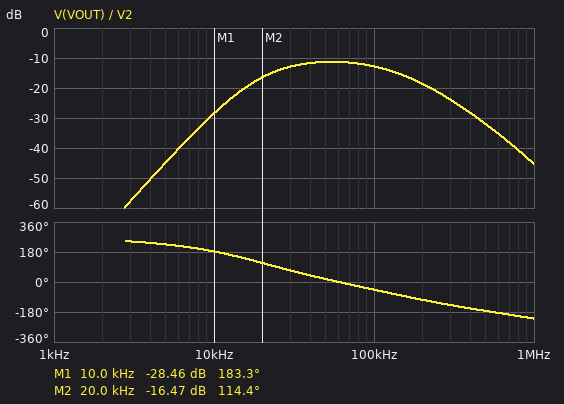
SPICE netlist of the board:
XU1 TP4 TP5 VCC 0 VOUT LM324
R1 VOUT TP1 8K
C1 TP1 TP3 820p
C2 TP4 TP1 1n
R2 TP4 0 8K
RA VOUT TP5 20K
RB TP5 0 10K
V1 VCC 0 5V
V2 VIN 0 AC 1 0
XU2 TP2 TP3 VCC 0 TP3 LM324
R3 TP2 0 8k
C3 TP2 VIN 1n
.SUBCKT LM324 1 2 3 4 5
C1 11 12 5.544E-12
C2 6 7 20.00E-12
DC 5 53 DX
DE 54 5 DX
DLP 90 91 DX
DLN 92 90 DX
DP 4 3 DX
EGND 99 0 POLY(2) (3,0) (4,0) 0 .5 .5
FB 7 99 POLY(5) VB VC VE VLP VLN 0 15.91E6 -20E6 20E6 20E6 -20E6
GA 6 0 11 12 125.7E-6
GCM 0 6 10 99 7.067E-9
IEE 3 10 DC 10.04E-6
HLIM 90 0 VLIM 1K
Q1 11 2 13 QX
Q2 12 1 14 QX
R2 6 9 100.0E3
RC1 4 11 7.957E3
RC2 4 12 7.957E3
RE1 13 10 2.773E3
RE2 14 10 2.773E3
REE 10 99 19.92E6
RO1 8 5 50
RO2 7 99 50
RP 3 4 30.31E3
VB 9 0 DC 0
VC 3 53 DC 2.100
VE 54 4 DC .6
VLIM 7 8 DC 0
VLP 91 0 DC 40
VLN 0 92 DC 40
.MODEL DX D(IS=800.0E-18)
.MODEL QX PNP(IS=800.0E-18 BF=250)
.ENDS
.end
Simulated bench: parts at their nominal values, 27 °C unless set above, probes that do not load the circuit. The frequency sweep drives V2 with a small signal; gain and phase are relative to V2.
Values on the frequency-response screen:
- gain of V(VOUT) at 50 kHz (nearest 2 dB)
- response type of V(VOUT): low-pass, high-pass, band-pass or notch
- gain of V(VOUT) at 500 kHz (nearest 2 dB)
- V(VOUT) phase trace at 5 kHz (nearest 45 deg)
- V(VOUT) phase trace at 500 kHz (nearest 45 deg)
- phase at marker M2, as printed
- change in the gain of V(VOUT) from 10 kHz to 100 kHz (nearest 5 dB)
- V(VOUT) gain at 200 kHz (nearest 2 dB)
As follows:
-12 dB
band-pass
-32 dB
225 deg
-180 deg
114.4 deg
15 dB
-18 dB
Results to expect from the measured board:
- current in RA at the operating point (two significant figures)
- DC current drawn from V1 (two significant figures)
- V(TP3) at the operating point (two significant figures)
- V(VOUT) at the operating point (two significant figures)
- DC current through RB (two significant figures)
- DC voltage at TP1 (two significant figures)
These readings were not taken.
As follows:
1.6 µA
350 µA
30 mV
47 mV
1.6 µA
47 mV
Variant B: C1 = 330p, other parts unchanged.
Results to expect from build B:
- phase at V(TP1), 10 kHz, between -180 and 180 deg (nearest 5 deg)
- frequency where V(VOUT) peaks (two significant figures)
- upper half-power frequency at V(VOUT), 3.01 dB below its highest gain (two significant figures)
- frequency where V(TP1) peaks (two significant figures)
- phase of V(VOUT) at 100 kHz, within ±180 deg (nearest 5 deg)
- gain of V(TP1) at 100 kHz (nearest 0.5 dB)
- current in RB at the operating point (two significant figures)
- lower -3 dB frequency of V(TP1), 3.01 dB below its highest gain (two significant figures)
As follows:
140 deg
63 kHz
150 kHz
96 kHz
-30 deg
-13.0 dB
1.6 µA
29 kHz
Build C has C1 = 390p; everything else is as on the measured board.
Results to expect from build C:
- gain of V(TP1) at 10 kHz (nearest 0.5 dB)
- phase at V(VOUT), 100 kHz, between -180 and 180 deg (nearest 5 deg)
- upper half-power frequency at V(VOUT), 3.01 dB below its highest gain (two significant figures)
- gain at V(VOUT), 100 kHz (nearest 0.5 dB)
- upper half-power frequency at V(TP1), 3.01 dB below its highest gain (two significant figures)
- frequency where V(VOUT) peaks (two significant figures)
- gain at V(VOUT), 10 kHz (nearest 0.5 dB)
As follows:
-28.0 dB
-35 deg
140 kHz
-14.5 dB
290 kHz
61 kHz
-34.5 dB
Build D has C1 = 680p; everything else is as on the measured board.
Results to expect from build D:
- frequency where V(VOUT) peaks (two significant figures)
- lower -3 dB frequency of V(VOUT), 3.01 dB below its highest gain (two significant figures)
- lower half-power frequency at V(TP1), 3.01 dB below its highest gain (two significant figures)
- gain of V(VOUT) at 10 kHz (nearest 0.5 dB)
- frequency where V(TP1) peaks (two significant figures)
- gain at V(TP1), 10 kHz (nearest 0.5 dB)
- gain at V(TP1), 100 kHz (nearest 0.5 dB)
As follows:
56 kHz
26 kHz
23 kHz
-30.0 dB
70 kHz
-23.5 dB
-11.0 dB
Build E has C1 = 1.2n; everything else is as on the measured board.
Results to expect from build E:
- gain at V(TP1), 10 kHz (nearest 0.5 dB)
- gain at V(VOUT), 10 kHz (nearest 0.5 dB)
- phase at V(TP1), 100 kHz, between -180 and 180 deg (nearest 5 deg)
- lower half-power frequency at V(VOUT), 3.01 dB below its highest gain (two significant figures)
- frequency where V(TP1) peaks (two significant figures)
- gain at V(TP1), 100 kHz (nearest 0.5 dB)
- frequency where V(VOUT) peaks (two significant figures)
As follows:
-19.5 dB
-26.0 dB
-15 deg
23 kHz
60 kHz
-10.0 dB
52 kHz
